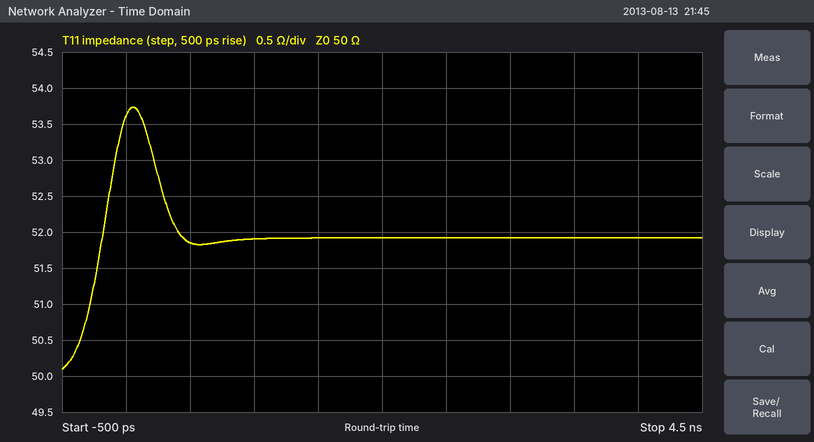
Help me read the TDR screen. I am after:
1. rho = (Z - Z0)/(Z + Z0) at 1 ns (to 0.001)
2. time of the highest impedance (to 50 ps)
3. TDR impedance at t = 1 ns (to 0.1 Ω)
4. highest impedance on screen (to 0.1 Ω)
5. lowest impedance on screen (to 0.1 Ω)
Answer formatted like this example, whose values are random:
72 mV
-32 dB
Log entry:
+0.019
50 ps
51.9 Ω
53.7 Ω
50.1 Ω
